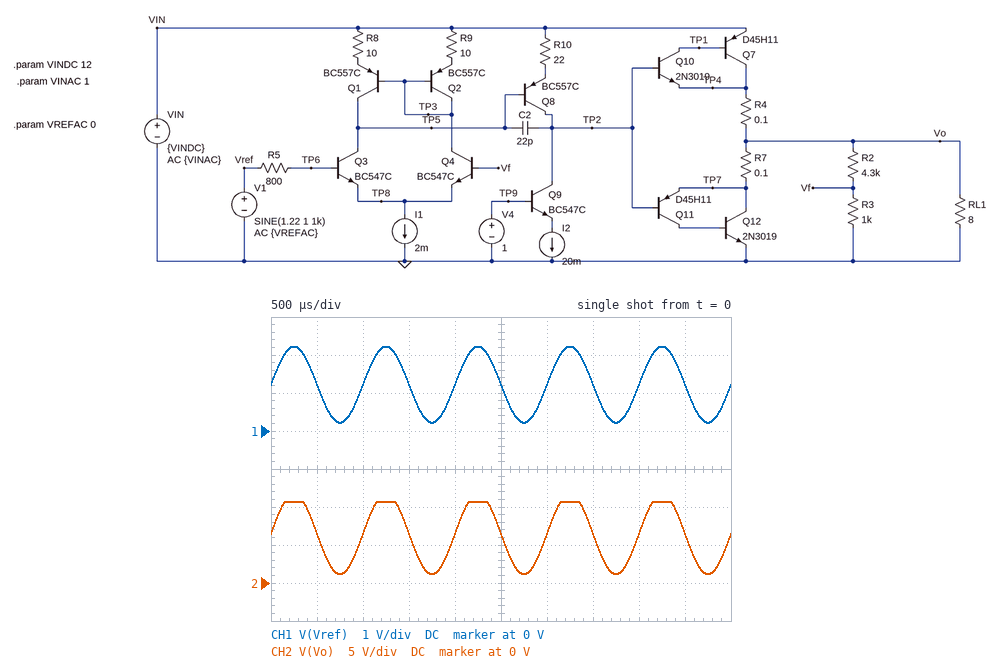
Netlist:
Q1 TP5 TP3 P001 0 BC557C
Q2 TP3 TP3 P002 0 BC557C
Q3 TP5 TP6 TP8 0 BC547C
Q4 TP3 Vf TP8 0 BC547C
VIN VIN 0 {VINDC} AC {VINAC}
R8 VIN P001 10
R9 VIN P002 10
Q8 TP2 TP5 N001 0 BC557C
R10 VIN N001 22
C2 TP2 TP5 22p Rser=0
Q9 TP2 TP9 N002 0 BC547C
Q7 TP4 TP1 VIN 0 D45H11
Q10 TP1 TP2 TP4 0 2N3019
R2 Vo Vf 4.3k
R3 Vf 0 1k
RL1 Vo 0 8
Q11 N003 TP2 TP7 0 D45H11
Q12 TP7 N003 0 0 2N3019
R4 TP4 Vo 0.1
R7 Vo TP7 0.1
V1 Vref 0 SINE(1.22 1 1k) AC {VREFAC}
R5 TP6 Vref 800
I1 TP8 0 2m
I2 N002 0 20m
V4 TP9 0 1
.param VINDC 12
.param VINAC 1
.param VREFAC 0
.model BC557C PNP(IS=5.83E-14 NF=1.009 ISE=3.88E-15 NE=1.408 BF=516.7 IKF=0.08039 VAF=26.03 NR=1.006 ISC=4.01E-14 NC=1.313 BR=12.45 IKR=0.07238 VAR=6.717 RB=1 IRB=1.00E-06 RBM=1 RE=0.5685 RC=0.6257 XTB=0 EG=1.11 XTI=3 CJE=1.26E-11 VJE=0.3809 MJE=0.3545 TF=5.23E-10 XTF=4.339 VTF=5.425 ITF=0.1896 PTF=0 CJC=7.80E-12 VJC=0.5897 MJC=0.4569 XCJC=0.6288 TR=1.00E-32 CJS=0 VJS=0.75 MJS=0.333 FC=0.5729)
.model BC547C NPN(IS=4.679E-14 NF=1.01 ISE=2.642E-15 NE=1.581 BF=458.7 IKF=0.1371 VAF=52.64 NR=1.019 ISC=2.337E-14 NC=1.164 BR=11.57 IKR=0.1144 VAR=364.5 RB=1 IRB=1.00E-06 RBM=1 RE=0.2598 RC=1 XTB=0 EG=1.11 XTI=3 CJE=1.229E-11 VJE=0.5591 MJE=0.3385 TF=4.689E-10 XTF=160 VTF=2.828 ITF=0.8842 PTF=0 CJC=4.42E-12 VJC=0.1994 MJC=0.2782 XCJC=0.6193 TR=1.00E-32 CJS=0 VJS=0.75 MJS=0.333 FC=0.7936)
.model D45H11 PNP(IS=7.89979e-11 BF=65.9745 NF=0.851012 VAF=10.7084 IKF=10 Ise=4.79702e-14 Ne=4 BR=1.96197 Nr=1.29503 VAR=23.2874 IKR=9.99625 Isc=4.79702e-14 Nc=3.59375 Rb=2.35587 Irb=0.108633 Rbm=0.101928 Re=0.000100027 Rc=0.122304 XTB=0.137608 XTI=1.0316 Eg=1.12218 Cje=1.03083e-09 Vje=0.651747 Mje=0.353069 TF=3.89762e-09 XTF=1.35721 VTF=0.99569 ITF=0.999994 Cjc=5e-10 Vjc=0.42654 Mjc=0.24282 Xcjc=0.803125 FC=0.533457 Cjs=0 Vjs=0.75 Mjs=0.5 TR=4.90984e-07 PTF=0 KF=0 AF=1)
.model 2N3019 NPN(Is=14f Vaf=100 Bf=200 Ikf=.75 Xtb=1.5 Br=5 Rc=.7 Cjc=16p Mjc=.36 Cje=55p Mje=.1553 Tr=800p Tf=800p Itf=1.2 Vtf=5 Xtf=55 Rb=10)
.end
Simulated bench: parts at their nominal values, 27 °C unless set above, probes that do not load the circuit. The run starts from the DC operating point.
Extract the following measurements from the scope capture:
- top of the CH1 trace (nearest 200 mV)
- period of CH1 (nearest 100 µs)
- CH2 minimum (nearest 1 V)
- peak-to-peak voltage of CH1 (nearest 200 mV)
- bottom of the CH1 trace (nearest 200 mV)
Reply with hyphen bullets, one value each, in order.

- 2.2 V
- 1.0 ms
- 1 V
- 2.0 V
- 200 mV
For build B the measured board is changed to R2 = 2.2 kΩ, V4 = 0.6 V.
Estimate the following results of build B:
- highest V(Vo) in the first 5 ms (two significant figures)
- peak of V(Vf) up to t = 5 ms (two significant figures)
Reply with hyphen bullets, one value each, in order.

- 7.1 V
- 2.2 V
